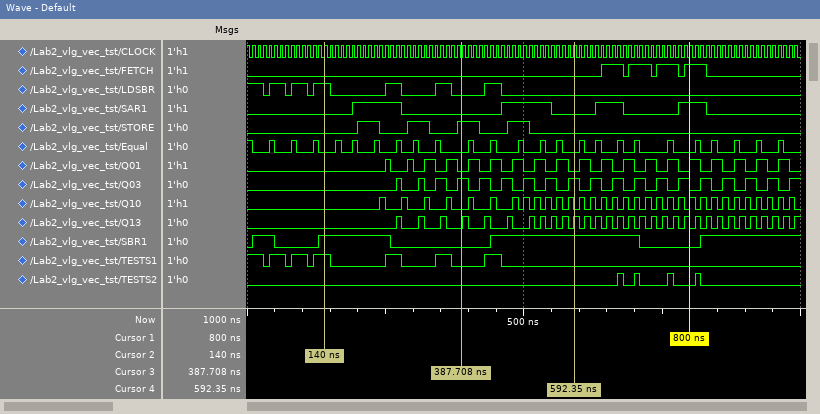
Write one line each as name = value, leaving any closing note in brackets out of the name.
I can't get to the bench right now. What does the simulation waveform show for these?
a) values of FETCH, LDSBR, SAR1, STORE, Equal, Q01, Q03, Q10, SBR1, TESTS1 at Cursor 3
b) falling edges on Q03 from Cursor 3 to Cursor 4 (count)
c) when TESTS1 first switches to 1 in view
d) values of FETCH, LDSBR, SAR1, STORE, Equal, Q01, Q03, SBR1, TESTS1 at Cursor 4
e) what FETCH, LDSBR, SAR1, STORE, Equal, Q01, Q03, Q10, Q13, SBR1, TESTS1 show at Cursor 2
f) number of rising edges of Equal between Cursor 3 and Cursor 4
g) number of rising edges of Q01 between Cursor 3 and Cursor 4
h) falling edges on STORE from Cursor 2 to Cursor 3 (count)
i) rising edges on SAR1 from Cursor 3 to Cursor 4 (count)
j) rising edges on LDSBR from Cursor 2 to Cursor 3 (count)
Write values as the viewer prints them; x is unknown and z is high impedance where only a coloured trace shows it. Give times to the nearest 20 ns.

values of FETCH, LDSBR, SAR1, STORE, Equal, Q01, Q03, Q10, SBR1, TESTS1 at Cursor 3 = FETCH=0, LDSBR=0, SAR1=0, STORE=1, Equal=0, Q01=0, Q03=1, Q10=0, SBR1=0, TESTS1=0
falling edges on Q03 from Cursor 3 to Cursor 4 = 5
when TESTS1 first switches to 1 in view = 40 ns
values of FETCH, LDSBR, SAR1, STORE, Equal, Q01, Q03, SBR1, TESTS1 at Cursor 4 = FETCH=0, LDSBR=0, SAR1=0, STORE=0, Equal=0, Q01=0, Q03=1, SBR1=1, TESTS1=0
what FETCH, LDSBR, SAR1, STORE, Equal, Q01, Q03, Q10, Q13, SBR1, TESTS1 show at Cursor 2 = FETCH=0, LDSBR=1, SAR1=0, STORE=0, Equal=0, Q01=0, Q03=0, Q10=0, Q13=0, SBR1=1, TESTS1=1
number of rising edges of Equal between Cursor 3 and Cursor 4 = 5
number of rising edges of Q01 between Cursor 3 and Cursor 4 = 5
falling edges on STORE from Cursor 2 to Cursor 3 = 2
rising edges on SAR1 from Cursor 3 to Cursor 4 = 1
rising edges on LDSBR from Cursor 2 to Cursor 3 = 2
